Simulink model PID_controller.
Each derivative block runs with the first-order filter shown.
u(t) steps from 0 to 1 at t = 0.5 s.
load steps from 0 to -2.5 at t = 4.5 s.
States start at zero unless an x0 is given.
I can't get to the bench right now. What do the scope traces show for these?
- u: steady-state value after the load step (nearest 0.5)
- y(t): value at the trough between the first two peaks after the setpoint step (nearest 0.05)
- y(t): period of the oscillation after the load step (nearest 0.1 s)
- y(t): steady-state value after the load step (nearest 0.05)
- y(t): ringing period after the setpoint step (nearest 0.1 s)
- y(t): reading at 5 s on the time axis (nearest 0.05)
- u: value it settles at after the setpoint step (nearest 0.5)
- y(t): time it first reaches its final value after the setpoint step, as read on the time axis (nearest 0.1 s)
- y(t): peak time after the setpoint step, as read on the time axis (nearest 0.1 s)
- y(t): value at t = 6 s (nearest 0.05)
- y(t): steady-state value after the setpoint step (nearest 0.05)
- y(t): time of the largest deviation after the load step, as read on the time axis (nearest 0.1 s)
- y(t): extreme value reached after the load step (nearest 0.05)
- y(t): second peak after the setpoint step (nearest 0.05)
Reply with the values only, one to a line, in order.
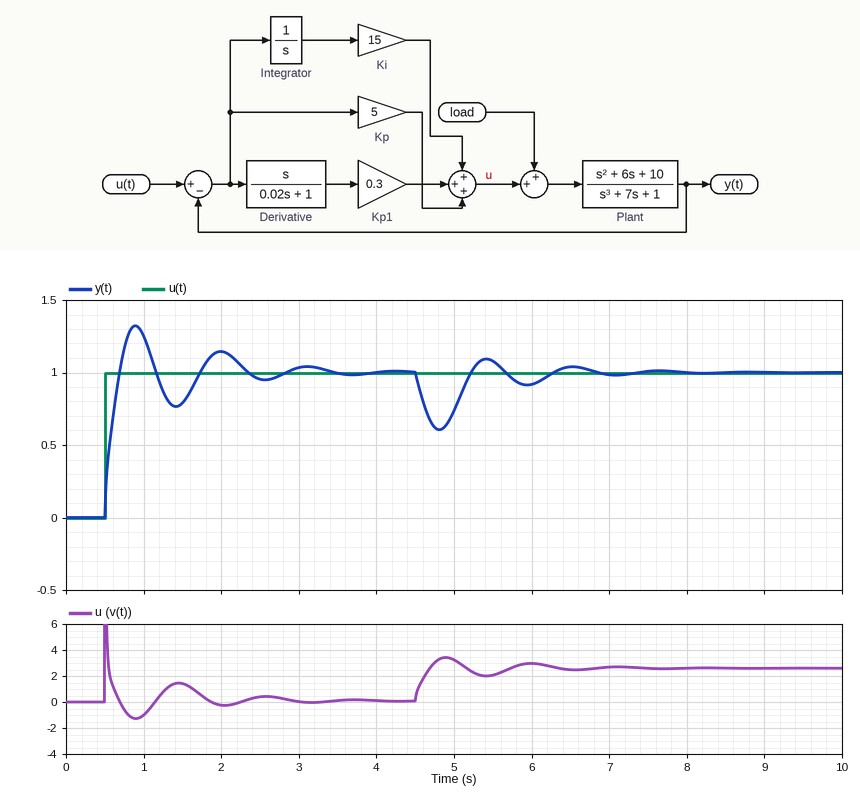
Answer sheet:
2.5
0.75
1.1 s
1.00
1.1 s
0.75
0.0
0.7 s
0.9 s
0.90
1.00
4.8 s
0.60
1.15
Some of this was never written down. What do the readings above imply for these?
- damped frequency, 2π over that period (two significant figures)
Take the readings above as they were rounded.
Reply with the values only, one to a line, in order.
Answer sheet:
5.7 rad/s
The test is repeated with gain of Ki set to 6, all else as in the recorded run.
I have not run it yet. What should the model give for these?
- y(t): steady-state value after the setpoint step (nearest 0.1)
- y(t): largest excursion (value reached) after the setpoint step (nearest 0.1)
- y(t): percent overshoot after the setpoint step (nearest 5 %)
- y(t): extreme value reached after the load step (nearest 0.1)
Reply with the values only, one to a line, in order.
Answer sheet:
1.0
1.2
25 %
0.5
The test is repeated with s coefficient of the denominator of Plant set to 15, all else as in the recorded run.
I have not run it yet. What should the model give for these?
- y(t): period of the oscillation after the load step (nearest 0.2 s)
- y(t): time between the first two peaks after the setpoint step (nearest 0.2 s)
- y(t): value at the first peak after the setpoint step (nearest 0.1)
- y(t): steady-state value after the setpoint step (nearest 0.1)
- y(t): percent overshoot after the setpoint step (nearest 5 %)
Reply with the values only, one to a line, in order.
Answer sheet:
1.0 s
1.0 s
1.2
1.0
20 %
